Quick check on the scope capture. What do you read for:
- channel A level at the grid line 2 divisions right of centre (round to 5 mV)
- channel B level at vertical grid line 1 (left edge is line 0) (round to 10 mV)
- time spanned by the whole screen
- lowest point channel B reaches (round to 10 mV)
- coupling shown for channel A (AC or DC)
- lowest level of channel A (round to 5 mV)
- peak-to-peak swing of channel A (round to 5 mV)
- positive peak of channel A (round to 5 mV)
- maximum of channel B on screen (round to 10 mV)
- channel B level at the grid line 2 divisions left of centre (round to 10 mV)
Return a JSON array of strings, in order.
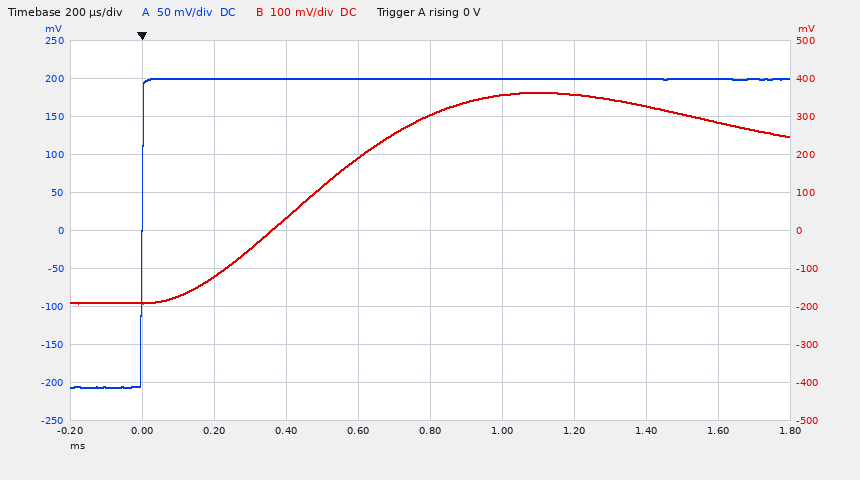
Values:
["200 mV", "-190 mV", "2 ms", "-190 mV", "DC", "-205 mV", "405 mV", "200 mV", "360 mV", "30 mV"]
